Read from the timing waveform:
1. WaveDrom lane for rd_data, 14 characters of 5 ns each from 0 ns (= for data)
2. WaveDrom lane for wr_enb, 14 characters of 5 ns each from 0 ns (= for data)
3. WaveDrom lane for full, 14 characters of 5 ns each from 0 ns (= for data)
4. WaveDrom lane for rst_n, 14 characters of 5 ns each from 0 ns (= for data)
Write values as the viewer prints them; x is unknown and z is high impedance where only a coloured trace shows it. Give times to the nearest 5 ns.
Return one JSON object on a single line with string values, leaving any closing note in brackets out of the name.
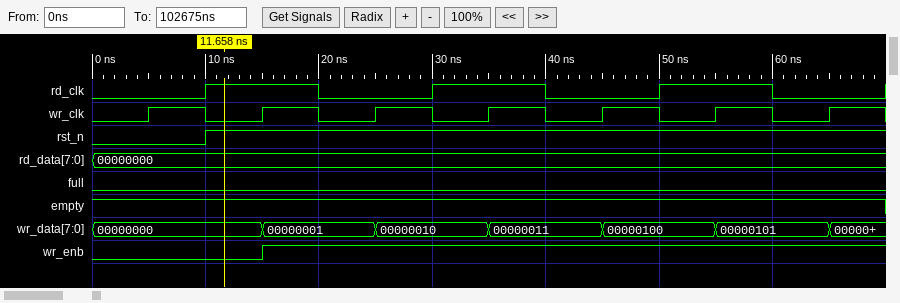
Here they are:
{"WaveDrom lane for rd_data, 14 characters of 5 ns each from 0 ns": "{name: 'rd_data', wave: '=.............', data: '00000000'}", "WaveDrom lane for wr_enb, 14 characters of 5 ns each from 0 ns": "{name: 'wr_enb', wave: '0..1..........'}", "WaveDrom lane for full, 14 characters of 5 ns each from 0 ns": "{name: 'full', wave: '0.............'}", "WaveDrom lane for rst_n, 14 characters of 5 ns each from 0 ns": "{name: 'rst_n', wave: '0.1...........'}"}
